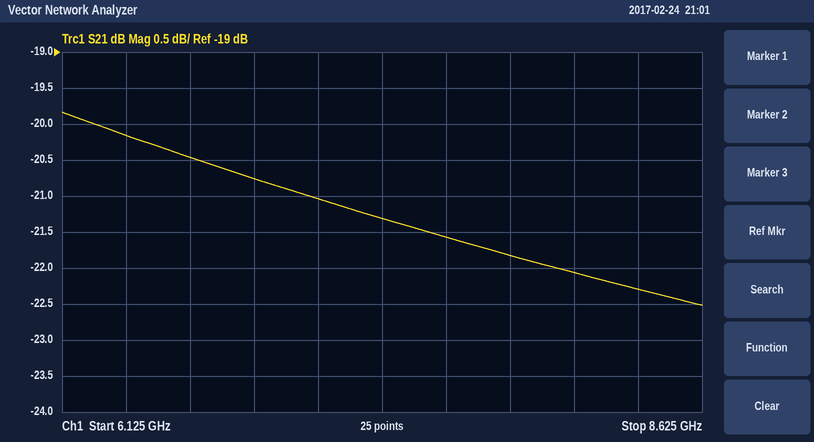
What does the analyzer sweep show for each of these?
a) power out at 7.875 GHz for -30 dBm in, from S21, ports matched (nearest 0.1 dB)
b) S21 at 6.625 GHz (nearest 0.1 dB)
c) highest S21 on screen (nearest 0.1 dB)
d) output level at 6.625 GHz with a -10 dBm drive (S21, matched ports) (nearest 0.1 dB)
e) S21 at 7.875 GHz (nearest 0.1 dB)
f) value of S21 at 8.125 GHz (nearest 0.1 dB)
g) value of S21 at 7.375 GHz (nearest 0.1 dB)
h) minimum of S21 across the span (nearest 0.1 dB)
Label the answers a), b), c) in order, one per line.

a) -51.8 dBm
b) -20.5 dB
c) -19.8 dB
d) -30.5 dBm
e) -21.8 dB
f) -22.1 dB
g) -21.3 dB
h) -22.5 dB
